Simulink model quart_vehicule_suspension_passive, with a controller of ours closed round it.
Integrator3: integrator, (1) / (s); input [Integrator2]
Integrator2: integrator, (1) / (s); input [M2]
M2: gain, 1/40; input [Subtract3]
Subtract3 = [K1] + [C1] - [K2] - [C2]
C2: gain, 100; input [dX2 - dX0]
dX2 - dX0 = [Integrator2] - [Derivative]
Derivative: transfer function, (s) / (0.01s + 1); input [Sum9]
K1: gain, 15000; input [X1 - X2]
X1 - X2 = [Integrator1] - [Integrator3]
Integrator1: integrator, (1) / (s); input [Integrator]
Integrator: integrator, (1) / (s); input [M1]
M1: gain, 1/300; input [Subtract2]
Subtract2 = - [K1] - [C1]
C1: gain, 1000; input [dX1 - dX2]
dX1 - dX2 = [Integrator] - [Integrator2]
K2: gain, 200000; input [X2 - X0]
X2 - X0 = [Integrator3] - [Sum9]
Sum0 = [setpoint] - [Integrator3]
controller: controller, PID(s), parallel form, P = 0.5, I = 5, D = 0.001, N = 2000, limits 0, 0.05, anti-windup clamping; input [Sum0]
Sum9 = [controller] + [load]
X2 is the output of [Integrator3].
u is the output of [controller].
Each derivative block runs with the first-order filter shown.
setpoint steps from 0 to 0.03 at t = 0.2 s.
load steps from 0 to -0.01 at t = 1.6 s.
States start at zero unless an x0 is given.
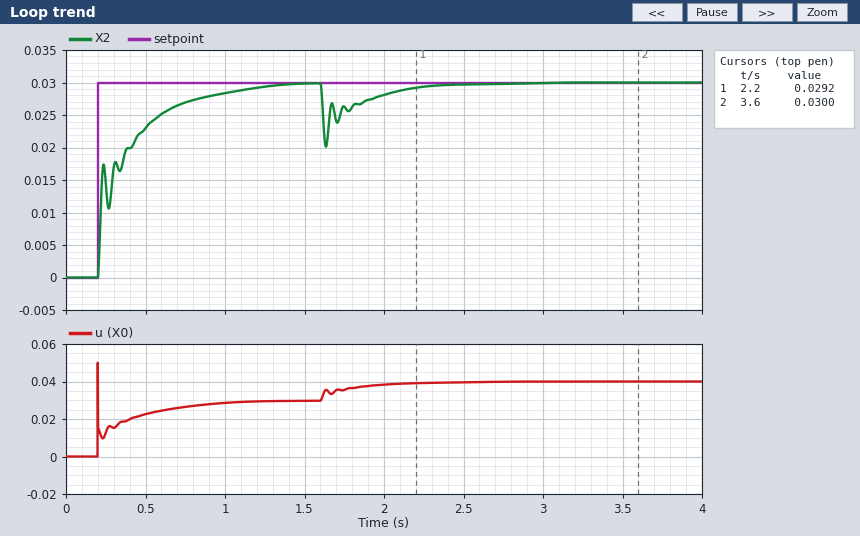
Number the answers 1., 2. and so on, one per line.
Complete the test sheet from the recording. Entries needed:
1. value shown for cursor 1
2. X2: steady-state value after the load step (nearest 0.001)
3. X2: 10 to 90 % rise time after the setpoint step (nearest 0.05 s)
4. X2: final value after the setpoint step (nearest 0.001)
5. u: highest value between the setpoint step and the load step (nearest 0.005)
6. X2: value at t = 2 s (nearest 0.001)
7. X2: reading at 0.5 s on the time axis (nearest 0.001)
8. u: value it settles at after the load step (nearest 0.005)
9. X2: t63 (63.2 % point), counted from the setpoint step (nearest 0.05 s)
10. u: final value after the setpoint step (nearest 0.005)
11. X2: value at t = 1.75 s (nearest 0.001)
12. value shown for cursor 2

1. 0.0292
2. 0.030
3. 0.55 s
4. 0.030
5. 0.050
6. 0.028
7. 0.023
8. 0.040
9. 0.15 s
10. 0.030
11. 0.026
12. 0.0300
